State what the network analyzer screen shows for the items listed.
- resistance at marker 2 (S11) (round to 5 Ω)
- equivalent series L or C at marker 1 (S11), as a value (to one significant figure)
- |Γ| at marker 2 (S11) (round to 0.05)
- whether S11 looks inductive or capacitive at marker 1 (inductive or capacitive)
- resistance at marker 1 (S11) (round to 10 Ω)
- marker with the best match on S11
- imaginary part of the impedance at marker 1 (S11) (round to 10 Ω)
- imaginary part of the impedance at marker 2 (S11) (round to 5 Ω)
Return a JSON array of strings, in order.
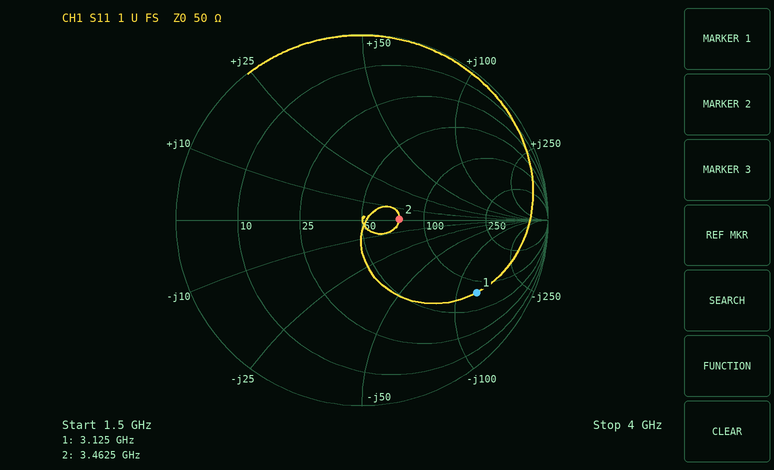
["75 Ω", "400 fF", "0.20", "capacitive", "80 Ω", "marker 2", "-130 Ω", "0 Ω"]
